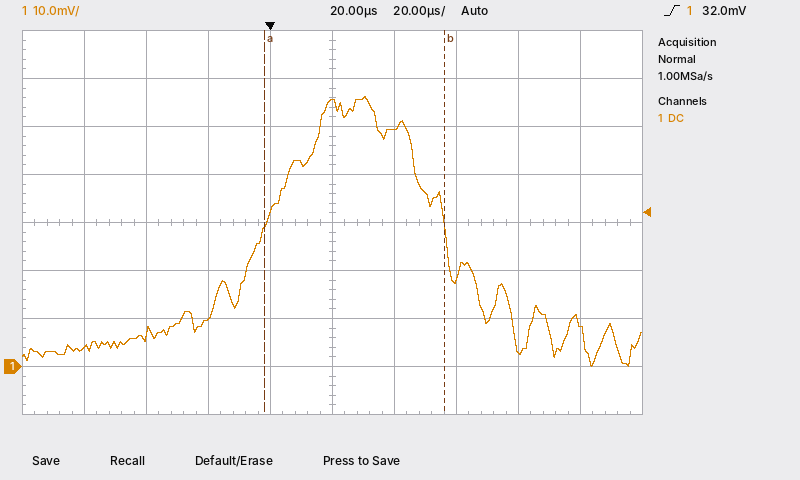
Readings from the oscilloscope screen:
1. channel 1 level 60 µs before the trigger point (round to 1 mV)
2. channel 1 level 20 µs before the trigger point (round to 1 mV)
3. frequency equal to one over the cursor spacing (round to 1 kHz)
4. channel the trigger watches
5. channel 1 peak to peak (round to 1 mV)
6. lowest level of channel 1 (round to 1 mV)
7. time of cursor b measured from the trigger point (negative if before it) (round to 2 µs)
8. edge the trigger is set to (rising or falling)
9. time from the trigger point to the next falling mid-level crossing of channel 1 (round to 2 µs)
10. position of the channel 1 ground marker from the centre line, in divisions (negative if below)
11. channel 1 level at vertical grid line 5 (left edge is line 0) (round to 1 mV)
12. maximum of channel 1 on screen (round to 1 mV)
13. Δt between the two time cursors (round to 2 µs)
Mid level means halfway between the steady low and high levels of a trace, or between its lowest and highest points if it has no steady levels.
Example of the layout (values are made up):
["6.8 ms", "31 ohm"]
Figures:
["4 mV", "10 mV", "17 kHz", "channel 1", "56 mV", "0 mV", "+56 µs", "rising", "56 µs", "-3.0 div", "55 mV", "56 mV", "58 µs"]
